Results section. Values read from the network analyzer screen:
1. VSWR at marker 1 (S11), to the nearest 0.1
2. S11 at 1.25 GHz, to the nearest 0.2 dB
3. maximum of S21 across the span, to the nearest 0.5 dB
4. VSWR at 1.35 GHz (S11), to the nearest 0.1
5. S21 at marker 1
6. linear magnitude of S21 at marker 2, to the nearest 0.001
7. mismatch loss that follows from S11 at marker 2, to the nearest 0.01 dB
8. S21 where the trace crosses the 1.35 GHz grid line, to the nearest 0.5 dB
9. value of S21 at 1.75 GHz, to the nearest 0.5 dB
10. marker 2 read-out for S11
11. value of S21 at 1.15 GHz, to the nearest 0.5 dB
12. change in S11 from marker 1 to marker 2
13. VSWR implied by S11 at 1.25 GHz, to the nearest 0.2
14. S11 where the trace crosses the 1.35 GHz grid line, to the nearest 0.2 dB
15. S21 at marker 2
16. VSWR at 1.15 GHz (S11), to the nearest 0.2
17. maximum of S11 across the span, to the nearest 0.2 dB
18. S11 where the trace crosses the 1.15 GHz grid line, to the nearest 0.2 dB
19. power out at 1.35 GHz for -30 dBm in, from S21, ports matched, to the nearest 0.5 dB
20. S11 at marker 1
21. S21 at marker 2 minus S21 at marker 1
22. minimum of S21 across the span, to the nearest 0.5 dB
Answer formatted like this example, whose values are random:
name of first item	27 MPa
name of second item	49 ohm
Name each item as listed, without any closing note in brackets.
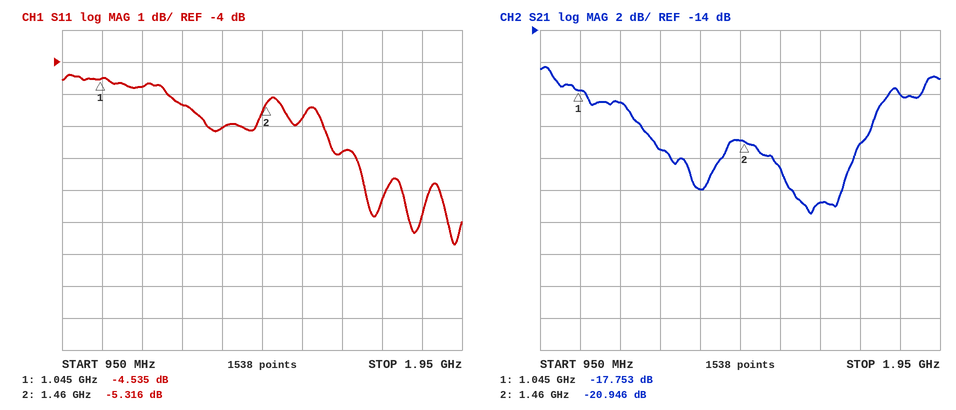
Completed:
VSWR at marker 1 (S11), to the nearest 0.1	3.9
S11 at 1.25 GHz, to the nearest 0.2 dB	-5.4 dB
maximum of S21 across the span, to the nearest 0.5 dB	-16.5 dB
VSWR at 1.35 GHz (S11), to the nearest 0.1	3.0
S21 at marker 1	-17.753 dB
linear magnitude of S21 at marker 2, to the nearest 0.001	0.090
mismatch loss that follows from S11 at marker 2, to the nearest 0.01 dB	1.51 dB
S21 where the trace crosses the 1.35 GHz grid line, to the nearest 0.5 dB	-24.0 dB
value of S21 at 1.75 GHz, to the nearest 0.5 dB	-21.0 dB
marker 2 read-out for S11	-5.316 dB
value of S21 at 1.15 GHz, to the nearest 0.5 dB	-18.5 dB
change in S11 from marker 1 to marker 2	-0.781 dB
VSWR implied by S11 at 1.25 GHz, to the nearest 0.2	3.4
S11 where the trace crosses the 1.35 GHz grid line, to the nearest 0.2 dB	-6.0 dB
S21 at marker 2	-20.946 dB
VSWR at 1.15 GHz (S11), to the nearest 0.2	3.8
maximum of S11 across the span, to the nearest 0.2 dB	-4.4 dB
S11 where the trace crosses the 1.15 GHz grid line, to the nearest 0.2 dB	-4.8 dB
power out at 1.35 GHz for -30 dBm in, from S21, ports matched, to the nearest 0.5 dB	-54.0 dBm
S11 at marker 1	-4.535 dB
S21 at marker 2 minus S21 at marker 1	-3.193 dB
minimum of S21 across the span, to the nearest 0.5 dB	-25.5 dB
